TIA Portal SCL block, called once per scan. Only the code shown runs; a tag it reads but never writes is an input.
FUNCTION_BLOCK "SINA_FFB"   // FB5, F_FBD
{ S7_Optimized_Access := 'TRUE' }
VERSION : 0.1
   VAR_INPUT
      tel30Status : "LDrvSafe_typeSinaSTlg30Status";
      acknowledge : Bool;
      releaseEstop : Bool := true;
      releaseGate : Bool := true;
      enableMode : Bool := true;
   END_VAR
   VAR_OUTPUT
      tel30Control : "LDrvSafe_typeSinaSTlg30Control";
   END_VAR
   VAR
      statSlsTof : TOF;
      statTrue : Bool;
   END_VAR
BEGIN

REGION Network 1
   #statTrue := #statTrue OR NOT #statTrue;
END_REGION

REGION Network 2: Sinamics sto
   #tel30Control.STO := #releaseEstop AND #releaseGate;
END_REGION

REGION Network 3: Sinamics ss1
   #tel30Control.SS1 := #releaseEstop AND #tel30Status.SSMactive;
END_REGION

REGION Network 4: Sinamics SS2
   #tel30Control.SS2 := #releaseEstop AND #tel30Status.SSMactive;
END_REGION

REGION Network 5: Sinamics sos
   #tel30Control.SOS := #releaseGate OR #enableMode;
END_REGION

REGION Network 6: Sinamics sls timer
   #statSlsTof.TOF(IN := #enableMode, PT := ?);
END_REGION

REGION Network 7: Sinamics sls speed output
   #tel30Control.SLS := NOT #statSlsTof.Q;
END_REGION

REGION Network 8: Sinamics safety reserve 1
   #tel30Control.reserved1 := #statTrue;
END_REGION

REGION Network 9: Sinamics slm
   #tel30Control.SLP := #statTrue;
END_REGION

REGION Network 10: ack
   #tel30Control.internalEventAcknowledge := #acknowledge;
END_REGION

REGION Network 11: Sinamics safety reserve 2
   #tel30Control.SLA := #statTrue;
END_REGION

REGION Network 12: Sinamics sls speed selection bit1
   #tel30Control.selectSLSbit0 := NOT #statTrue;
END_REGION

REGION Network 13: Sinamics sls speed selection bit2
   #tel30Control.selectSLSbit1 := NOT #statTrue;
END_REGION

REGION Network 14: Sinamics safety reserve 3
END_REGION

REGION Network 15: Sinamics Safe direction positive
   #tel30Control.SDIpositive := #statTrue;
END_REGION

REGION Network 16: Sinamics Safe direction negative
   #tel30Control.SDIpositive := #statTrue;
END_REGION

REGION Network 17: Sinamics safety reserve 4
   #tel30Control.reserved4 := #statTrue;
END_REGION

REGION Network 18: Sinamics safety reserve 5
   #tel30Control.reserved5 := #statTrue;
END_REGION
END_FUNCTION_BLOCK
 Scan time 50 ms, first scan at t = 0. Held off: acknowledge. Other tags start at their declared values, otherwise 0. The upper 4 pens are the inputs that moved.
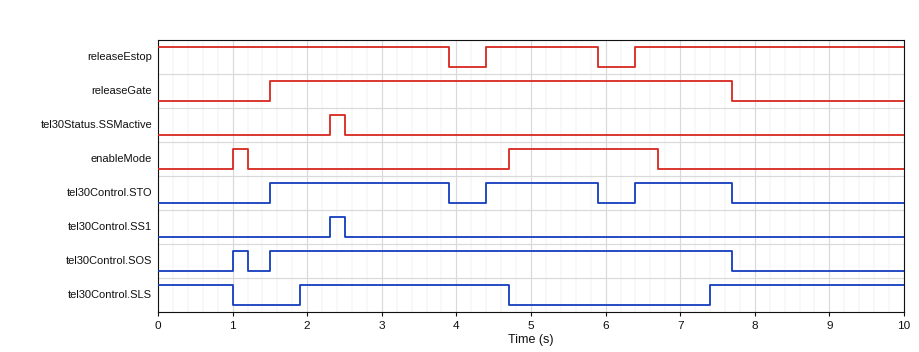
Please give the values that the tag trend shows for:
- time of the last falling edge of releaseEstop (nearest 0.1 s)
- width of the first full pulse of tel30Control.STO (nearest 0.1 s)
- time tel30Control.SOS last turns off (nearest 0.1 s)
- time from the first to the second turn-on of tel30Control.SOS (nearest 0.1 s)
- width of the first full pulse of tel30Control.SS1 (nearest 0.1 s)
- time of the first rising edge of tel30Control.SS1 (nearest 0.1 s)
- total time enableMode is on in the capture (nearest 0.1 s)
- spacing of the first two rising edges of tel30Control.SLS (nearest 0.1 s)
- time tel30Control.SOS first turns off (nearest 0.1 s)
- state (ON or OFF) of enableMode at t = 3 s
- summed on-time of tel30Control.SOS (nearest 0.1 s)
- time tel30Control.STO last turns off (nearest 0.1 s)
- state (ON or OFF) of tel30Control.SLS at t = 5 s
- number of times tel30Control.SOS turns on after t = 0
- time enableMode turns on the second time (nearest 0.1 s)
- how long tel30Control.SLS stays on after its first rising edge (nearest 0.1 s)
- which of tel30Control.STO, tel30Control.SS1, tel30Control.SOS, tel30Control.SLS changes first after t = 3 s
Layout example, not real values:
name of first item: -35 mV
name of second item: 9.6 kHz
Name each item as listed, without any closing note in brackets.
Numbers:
time of the last falling edge of releaseEstop: 5.9 s
width of the first full pulse of tel30Control.STO: 2.4 s
time tel30Control.SOS last turns off: 7.7 s
time from the first to the second turn-on of tel30Control.SOS: 0.5 s
width of the first full pulse of tel30Control.SS1: 0.2 s
time of the first rising edge of tel30Control.SS1: 2.3 s
total time enableMode is on in the capture: 2.2 s
spacing of the first two rising edges of tel30Control.SLS: 5.5 s
time tel30Control.SOS first turns off: 1.2 s
state (ON or OFF) of enableMode at t = 3 s: OFF
summed on-time of tel30Control.SOS: 6.4 s
time tel30Control.STO last turns off: 7.7 s
state (ON or OFF) of tel30Control.SLS at t = 5 s: OFF
number of times tel30Control.SOS turns on after t = 0: 2
time enableMode turns on the second time: 4.7 s
how long tel30Control.SLS stays on after its first rising edge: 2.8 s
which of tel30Control.STO, tel30Control.SS1, tel30Control.SOS, tel30Control.SLS changes first after t = 3 s: tel30Control.STO
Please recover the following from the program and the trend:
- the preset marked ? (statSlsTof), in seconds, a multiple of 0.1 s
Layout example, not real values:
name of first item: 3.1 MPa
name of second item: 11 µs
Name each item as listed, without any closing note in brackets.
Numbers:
the preset marked ? (statSlsTof), in seconds, a multiple of 0.1 s: 0.7 s
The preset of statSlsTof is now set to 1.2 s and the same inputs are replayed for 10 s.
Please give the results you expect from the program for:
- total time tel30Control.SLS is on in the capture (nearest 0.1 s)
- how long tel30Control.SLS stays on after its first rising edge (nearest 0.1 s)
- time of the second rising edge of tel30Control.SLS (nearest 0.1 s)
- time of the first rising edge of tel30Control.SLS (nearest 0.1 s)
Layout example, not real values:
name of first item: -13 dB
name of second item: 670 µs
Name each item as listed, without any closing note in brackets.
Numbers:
total time tel30Control.SLS is on in the capture: 5.4 s
how long tel30Control.SLS stays on after its first rising edge: 2.3 s
time of the second rising edge of tel30Control.SLS: 7.9 s
time of the first rising edge of tel30Control.SLS: 2.4 s
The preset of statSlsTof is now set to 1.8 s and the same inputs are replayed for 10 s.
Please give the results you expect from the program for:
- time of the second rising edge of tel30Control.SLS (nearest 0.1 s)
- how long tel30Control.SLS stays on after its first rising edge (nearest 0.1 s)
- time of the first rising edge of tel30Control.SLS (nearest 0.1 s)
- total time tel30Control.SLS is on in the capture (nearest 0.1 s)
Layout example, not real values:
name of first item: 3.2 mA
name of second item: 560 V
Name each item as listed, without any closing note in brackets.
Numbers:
time of the second rising edge of tel30Control.SLS: 8.5 s
how long tel30Control.SLS stays on after its first rising edge: 1.7 s
time of the first rising edge of tel30Control.SLS: 3.0 s
total time tel30Control.SLS is on in the capture: 4.2 s
